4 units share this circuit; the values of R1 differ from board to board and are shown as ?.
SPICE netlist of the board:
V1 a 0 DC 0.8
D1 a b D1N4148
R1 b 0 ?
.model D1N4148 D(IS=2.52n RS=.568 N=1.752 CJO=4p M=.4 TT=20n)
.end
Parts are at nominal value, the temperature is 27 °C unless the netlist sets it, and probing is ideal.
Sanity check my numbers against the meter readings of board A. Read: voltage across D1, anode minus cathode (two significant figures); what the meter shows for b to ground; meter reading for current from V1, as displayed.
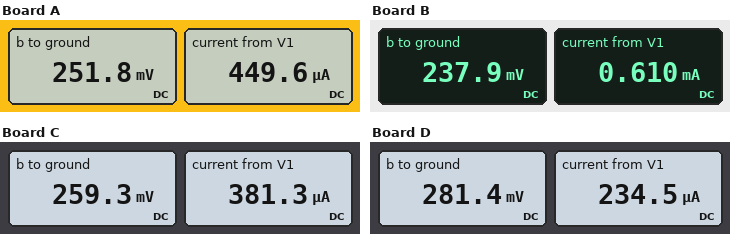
550 mV
251.8 mV
449.6 µA
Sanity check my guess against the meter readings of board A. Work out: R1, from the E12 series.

560 Ω
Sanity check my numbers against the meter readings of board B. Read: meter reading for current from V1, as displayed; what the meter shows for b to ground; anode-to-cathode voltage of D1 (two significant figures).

0.610 mA
237.9 mV
560 mV
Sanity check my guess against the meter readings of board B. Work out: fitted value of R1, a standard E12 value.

390 Ω
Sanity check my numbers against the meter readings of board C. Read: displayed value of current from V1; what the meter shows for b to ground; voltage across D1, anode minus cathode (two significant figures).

381.3 µA
259.3 mV
540 mV
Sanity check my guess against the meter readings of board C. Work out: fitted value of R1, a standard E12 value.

680 Ω
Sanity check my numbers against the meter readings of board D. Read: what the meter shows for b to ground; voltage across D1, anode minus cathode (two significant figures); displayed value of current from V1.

281.4 mV
520 mV
234.5 µA
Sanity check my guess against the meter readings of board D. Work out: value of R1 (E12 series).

1.2 kΩ
